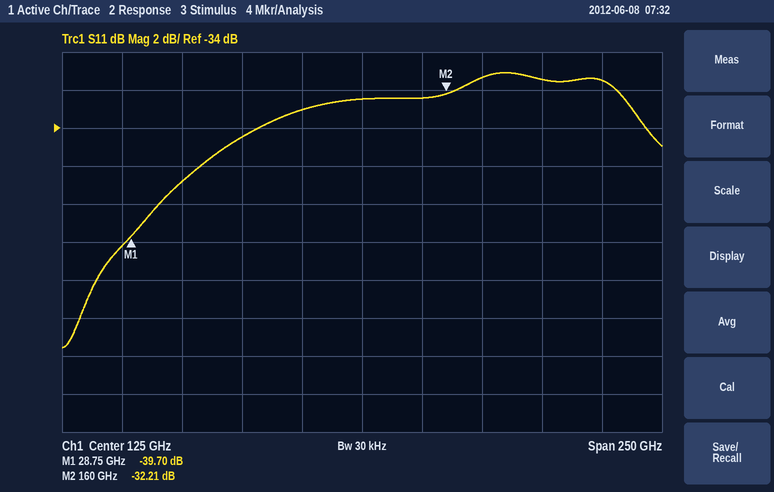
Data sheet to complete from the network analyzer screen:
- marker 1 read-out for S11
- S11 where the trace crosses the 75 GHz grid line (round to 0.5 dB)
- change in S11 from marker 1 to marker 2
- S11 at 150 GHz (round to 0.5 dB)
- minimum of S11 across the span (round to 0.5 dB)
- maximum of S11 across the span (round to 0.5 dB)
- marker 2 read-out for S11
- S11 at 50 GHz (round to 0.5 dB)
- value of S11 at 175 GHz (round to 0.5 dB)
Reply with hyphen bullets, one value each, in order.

- -39.70 dB
- -34.5 dB
- 7.49 dB
- -32.5 dB
- -45.5 dB
- -31.0 dB
- -32.21 dB
- -37.0 dB
- -31.5 dB
